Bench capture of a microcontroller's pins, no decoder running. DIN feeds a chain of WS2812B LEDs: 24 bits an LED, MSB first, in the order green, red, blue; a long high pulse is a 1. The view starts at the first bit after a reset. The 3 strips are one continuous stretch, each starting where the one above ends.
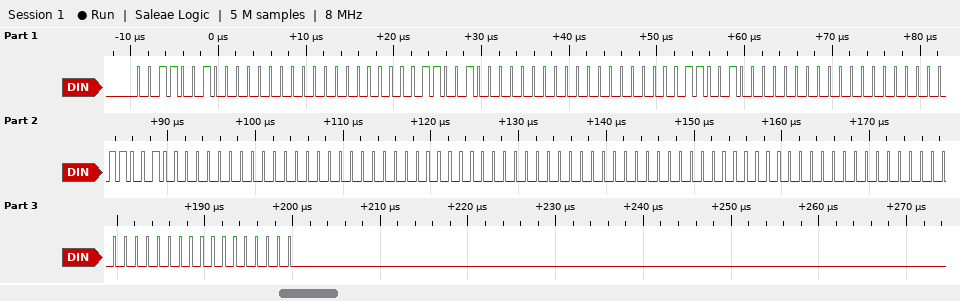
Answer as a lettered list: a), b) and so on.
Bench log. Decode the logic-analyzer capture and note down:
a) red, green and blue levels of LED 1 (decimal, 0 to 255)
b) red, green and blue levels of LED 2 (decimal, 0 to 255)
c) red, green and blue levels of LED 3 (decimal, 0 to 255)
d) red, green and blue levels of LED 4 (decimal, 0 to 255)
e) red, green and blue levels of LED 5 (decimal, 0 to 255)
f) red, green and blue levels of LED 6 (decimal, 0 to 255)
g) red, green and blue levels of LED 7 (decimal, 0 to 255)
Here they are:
a) 0, 50, 0
b) 0, 50, 0
c) 0, 50, 0
d) 0, 50, 0
e) 0, 0, 0
f) 0, 0, 0
g) 0, 0, 0
